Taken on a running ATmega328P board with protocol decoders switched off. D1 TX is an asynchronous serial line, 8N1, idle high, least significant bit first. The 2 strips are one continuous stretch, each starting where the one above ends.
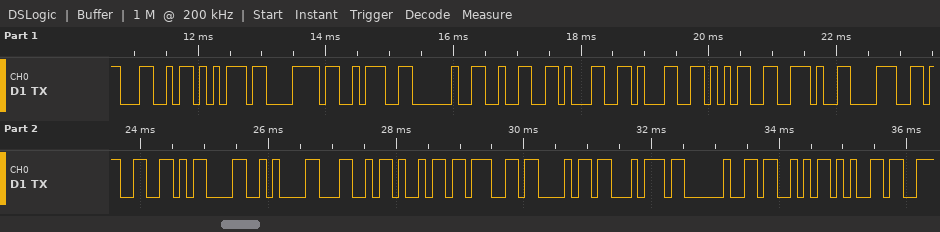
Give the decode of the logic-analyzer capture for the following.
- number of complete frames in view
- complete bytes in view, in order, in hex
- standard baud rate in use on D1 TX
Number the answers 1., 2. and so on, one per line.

1. 22
2. 4C 75 78 3A 20 32 31 31 35 2E 38 33 0D 0A 4C 69 67 68 74 20 53 65
3. 9600 baud
